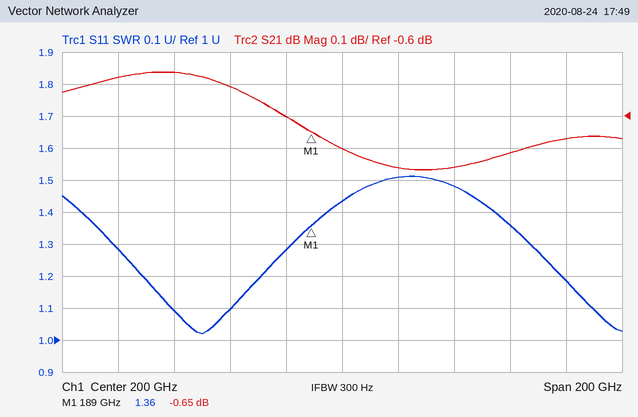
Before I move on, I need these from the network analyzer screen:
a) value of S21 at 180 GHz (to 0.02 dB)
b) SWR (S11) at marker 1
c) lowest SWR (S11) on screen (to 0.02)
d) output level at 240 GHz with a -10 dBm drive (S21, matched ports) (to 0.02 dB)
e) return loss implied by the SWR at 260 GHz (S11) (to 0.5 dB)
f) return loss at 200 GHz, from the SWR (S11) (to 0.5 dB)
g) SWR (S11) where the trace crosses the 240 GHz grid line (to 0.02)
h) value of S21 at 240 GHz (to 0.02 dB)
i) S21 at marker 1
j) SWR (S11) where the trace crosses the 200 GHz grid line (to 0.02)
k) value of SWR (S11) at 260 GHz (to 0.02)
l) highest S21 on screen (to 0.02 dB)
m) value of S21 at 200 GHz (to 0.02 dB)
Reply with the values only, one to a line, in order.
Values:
-0.60 dB
1.36
1.02
-10.76 dBm
16.5 dB
15.0 dB
1.48
-0.76 dB
-0.65 dB
1.44
1.36
-0.46 dB
-0.70 dB
